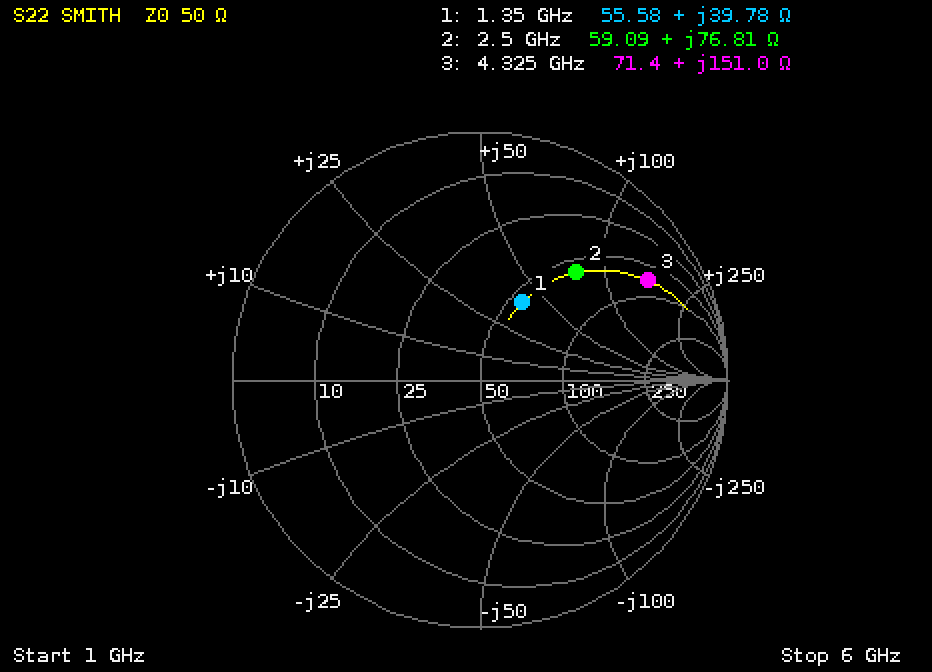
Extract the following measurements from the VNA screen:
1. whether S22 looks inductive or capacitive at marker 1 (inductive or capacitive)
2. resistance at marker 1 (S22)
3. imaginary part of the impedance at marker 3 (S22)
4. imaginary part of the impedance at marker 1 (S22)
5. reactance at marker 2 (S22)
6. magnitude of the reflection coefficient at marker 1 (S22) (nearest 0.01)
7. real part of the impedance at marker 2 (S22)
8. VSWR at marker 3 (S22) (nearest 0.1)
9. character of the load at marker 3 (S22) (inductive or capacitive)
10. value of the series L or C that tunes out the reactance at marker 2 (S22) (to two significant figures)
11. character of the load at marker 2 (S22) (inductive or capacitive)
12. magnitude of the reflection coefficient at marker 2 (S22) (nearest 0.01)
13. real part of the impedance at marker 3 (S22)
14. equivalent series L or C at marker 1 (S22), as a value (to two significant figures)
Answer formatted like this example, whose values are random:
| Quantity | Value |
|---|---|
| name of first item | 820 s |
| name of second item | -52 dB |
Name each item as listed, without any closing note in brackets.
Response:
| Quantity | Value |
|---|---|
| whether S22 looks inductive or capacitive at marker 1 | inductive |
| resistance at marker 1 | 55.58 Ω |
| imaginary part of the impedance at marker 3 | +151.0 Ω |
| imaginary part of the impedance at marker 1 | +39.78 Ω |
| reactance at marker 2 | +76.81 Ω |
| magnitude of the reflection coefficient at marker 1 (S22) | 0.36 |
| real part of the impedance at marker 2 | 59.09 Ω |
| VSWR at marker 3 (S22) | 8.4 |
| character of the load at marker 3 (S22) | inductive |
| value of the series L or C that tunes out the reactance at marker 2 (S22) | 830 fF |
| character of the load at marker 2 (S22) | inductive |
| magnitude of the reflection coefficient at marker 2 (S22) | 0.58 |
| real part of the impedance at marker 3 | 71.4 Ω |
| equivalent series L or C at marker 1 (S22), as a value | 4.7 nH |
